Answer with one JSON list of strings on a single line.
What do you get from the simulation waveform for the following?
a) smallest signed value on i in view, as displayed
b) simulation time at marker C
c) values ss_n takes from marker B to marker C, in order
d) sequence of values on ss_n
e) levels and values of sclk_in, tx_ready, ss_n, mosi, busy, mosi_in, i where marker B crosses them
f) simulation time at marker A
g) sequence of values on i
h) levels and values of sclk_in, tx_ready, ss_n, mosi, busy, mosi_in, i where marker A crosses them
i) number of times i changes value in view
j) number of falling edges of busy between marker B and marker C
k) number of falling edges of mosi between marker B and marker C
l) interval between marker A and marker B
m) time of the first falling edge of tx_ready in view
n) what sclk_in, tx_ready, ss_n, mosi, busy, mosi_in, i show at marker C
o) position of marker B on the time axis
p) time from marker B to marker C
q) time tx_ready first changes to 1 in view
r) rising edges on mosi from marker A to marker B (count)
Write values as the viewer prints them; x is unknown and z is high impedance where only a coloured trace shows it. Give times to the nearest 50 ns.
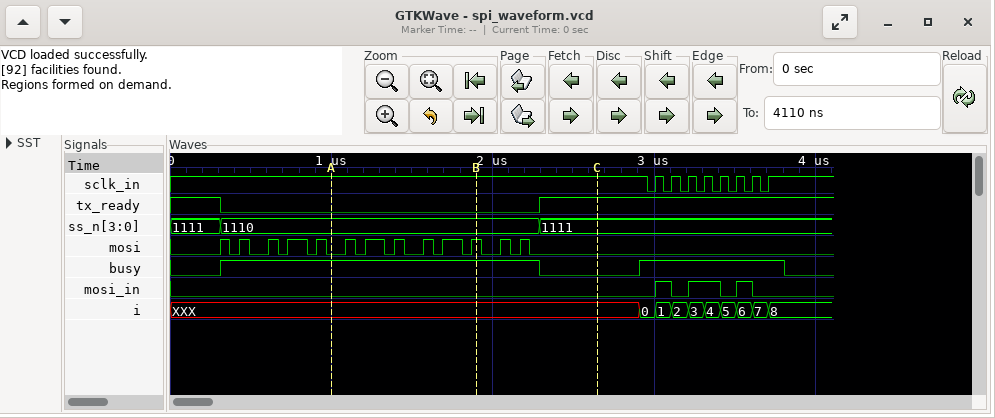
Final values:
["0", "2650 ns", "1110, 1111", "1111, 1110, 1111", "sclk_in=1, tx_ready=0, ss_n=1110, mosi=1, busy=1, mosi_in=0, i=XXX", "1000 ns", "XXX, 0, 1, 2, 3, 4, 5, 6, 7, 8", "sclk_in=1, tx_ready=0, ss_n=1110, mosi=0, busy=1, mosi_in=0, i=XXX", "9", "1", "3", "900 ns", "300 ns", "sclk_in=1, tx_ready=1, ss_n=1111, mosi=0, busy=0, mosi_in=0, i=XXX", "1900 ns", "750 ns", "2300 ns", "6"]
